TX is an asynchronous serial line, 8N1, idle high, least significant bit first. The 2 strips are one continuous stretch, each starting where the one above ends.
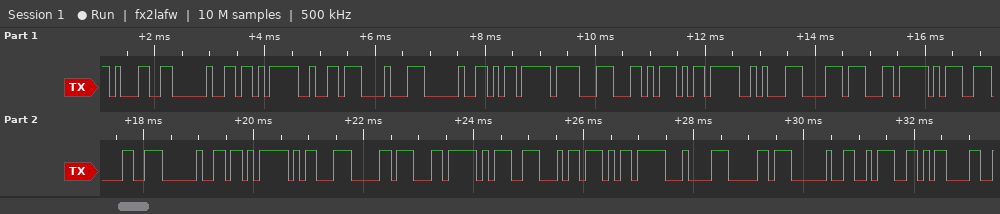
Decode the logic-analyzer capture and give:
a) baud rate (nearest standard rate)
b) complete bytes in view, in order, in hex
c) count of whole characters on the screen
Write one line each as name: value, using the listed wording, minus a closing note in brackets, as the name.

baud rate: 9600 baud
complete bytes in view, in order, in hex: 31 20 EB B2 88 20 ED 8F AC ED 8A B8 EC 9D 98 20 EB 8D B0 EC 9D B4 ED 84 B0 20 3A 0D
count of whole characters on the screen: 28
